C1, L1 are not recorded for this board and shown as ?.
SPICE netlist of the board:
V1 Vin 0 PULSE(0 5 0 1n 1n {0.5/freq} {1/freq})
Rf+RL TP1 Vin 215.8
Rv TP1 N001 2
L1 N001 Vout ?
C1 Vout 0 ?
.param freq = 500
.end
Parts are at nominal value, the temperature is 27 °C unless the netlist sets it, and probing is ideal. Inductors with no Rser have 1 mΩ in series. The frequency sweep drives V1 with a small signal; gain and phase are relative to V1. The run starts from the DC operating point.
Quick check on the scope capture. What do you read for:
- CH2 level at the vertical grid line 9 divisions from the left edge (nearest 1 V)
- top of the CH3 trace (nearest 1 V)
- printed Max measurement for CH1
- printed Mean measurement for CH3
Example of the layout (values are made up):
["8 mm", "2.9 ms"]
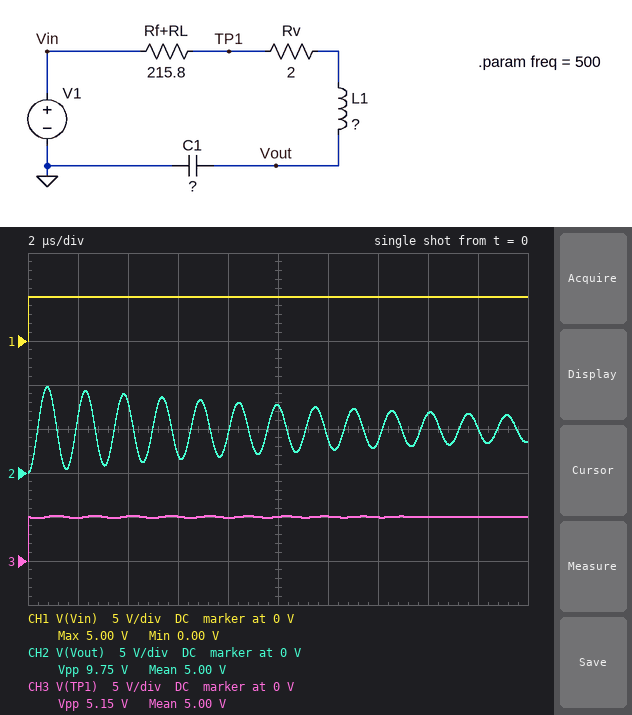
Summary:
["5 V", "5 V", "5.00 V", "5.00 V"]
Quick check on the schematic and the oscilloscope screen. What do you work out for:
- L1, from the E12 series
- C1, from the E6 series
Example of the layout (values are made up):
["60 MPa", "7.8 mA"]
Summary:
["1.8 mH", "33 pF"]
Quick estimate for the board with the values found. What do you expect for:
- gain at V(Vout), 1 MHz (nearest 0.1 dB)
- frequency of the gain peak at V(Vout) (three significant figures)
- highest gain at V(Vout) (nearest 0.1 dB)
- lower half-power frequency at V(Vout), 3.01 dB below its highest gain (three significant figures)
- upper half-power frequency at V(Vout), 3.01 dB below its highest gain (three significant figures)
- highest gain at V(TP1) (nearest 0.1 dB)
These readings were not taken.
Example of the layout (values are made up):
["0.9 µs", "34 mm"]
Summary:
["-2.6 dB", "653 kHz", "30.6 dB", "643 kHz", "662 kHz", "0 dB"]
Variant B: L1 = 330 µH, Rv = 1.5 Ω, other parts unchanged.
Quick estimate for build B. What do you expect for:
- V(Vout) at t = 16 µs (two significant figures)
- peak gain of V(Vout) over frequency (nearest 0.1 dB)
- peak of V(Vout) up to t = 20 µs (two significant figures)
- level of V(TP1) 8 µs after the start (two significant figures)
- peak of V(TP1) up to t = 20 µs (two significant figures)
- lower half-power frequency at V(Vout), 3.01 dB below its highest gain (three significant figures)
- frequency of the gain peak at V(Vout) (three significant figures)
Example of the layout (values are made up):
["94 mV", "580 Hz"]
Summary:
["5.0 V", "23.3 dB", "9.5 V", "5.0 V", "5.3 V", "1.47 MHz", "1.52 MHz"]
